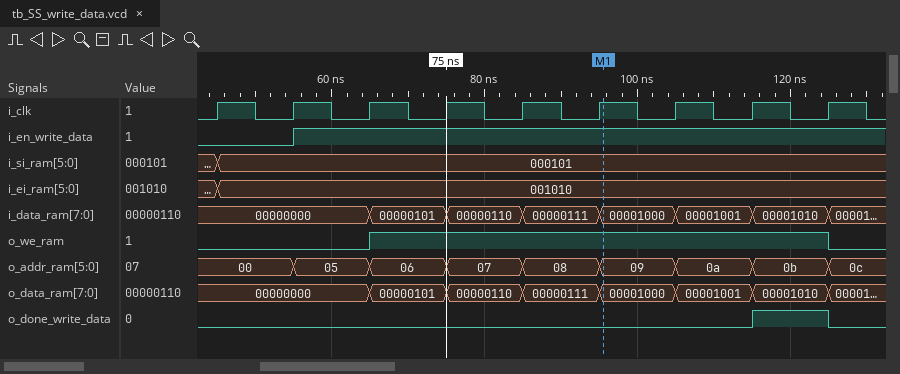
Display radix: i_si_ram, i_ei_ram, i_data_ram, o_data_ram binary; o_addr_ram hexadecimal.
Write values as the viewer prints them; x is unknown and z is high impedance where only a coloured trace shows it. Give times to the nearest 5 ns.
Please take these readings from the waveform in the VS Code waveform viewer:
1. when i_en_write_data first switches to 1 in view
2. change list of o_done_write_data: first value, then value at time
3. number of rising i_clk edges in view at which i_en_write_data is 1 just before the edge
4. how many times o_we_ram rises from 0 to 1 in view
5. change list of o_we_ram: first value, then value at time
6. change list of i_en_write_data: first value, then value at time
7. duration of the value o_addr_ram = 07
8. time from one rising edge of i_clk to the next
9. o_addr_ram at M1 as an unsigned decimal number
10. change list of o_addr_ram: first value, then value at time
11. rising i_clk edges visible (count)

55 ns
0, 1 at 115 ns, 0 at 125 ns
7
1
0, 1 at 65 ns, 0 at 125 ns
0, 1 at 55 ns
10 ns
10 ns
9
00, 05 at 55 ns, 06 at 65 ns, 07 at 75 ns, 08 at 85 ns, 09 at 95 ns, 0a at 105 ns, 0b at 115 ns, 0c at 125 ns
9
